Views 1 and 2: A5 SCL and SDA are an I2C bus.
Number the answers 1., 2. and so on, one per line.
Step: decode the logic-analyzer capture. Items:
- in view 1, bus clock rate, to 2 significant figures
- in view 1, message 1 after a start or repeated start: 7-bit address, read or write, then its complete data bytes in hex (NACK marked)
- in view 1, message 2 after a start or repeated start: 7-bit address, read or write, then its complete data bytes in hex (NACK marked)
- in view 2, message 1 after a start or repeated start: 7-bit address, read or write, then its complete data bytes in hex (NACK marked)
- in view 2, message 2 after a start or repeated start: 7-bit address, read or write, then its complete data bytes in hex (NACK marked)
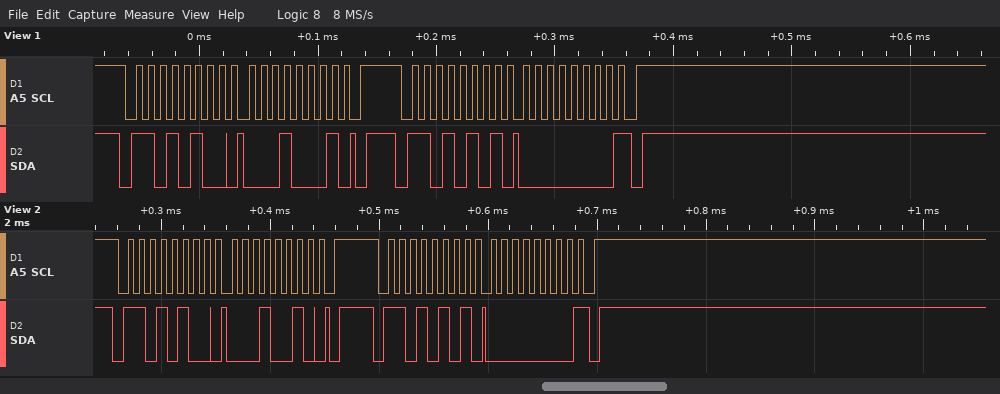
1. 100 kHz
2. 0x6A write: 11
3. 0x6A read: 00 NACK
4. 0x6A write: 12
5. 0x6A read: 00 NACK
